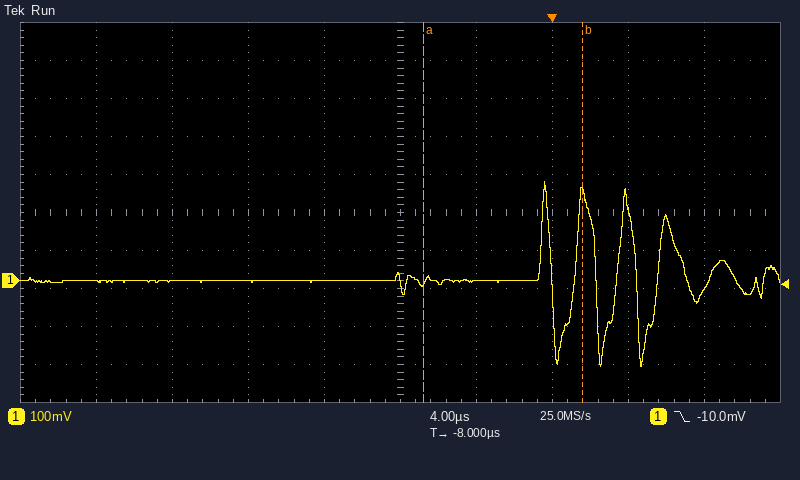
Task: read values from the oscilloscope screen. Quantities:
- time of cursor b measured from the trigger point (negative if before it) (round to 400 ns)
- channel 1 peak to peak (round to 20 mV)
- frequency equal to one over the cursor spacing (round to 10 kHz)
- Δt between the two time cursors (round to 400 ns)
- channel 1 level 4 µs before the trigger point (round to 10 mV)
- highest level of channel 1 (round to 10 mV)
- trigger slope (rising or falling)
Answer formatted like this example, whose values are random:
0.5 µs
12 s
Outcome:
+1.6 µs
480 mV
120 kHz
8.4 µs
0 mV
260 mV
falling
